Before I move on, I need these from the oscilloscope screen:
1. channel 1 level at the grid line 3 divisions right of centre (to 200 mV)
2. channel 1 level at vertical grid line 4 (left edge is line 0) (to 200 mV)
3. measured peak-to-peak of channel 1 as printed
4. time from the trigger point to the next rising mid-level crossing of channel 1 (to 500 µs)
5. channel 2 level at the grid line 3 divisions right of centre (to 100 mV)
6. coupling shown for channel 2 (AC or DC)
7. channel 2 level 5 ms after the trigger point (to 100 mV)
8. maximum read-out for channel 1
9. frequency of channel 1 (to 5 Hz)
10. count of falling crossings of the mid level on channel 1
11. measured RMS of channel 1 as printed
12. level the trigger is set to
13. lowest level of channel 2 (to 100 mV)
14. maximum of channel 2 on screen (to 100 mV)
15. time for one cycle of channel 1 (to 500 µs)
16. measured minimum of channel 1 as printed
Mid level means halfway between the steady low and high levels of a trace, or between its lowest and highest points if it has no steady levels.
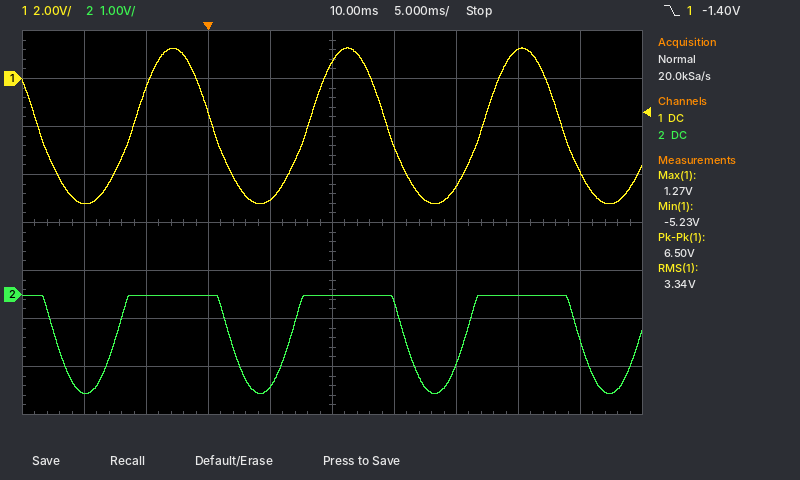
1.2 V
-5.0 V
6.50 V
8.0 ms
0.0 V
DC
-1.9 V
1.27 V
70 Hz
4
3.34 V
-1.40 V
-2.1 V
0.0 V
14.0 ms
-5.23 V
